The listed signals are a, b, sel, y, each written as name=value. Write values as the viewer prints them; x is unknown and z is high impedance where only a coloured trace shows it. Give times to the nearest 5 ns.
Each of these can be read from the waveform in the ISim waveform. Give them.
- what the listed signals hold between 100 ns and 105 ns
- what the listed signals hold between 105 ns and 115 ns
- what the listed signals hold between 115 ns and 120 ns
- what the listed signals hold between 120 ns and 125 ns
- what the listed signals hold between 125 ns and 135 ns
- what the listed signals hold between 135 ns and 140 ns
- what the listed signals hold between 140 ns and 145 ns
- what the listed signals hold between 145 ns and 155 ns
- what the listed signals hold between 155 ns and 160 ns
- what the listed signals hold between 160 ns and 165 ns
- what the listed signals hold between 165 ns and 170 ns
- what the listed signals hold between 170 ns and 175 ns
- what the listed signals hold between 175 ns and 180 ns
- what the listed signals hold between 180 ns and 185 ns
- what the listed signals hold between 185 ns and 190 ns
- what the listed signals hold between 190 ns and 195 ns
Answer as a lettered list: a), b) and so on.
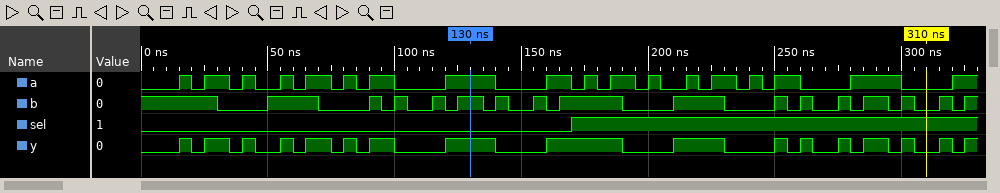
a) a=0, b=1, sel=0, y=0
b) a=0, b=0, sel=0, y=0
c) a=0, b=1, sel=0, y=0
d) a=1, b=0, sel=0, y=1
e) a=1, b=1, sel=0, y=1
f) a=1, b=0, sel=0, y=1
g) a=0, b=1, sel=0, y=0
h) a=0, b=0, sel=0, y=0
i) a=0, b=1, sel=0, y=0
j) a=1, b=0, sel=0, y=1
k) a=1, b=1, sel=0, y=1
l) a=0, b=1, sel=1, y=1
m) a=1, b=1, sel=1, y=1
n) a=0, b=1, sel=1, y=1
o) a=1, b=1, sel=1, y=1
p) a=1, b=0, sel=1, y=0
